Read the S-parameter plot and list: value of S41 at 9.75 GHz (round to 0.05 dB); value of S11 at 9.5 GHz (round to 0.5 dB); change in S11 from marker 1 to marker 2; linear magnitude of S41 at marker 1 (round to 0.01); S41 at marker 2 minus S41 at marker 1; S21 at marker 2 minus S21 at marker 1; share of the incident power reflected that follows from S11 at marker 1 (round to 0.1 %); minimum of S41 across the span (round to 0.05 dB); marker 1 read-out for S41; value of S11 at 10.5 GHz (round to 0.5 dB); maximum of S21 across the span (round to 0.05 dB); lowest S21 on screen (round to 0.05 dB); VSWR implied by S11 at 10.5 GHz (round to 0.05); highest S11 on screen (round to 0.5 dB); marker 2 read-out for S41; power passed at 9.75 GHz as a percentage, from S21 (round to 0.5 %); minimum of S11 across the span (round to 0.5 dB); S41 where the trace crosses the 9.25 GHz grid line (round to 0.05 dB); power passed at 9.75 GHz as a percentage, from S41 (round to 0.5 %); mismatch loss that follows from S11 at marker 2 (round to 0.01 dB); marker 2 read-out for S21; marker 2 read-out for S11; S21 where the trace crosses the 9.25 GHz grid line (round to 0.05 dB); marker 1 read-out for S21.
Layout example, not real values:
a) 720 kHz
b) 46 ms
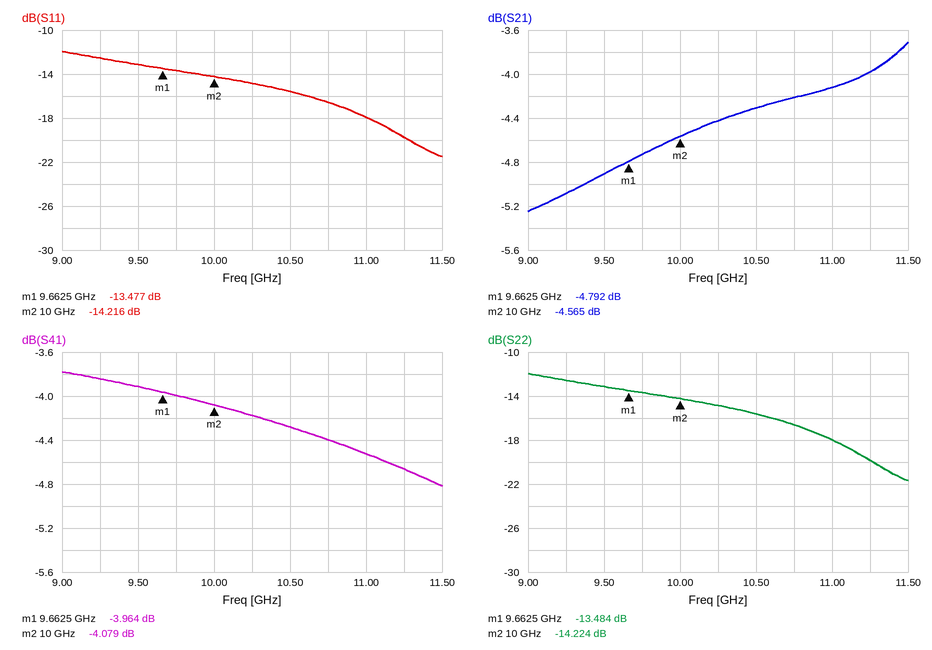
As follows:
a) -4.00 dB
b) -13.0 dB
c) -0.739 dB
d) 0.63
e) -0.115 dB
f) 0.227 dB
g) 4.5 %
h) -4.80 dB
i) -3.964 dB
j) -15.5 dB
k) -3.70 dB
l) -5.25 dB
m) 1.40
n) -12.0 dB
o) -4.079 dB
p) 33.5 %
q) -21.5 dB
r) -3.85 dB
s) 40.0 %
t) 0.17 dB
u) -4.565 dB
v) -14.216 dB
w) -5.10 dB
x) -4.792 dB
